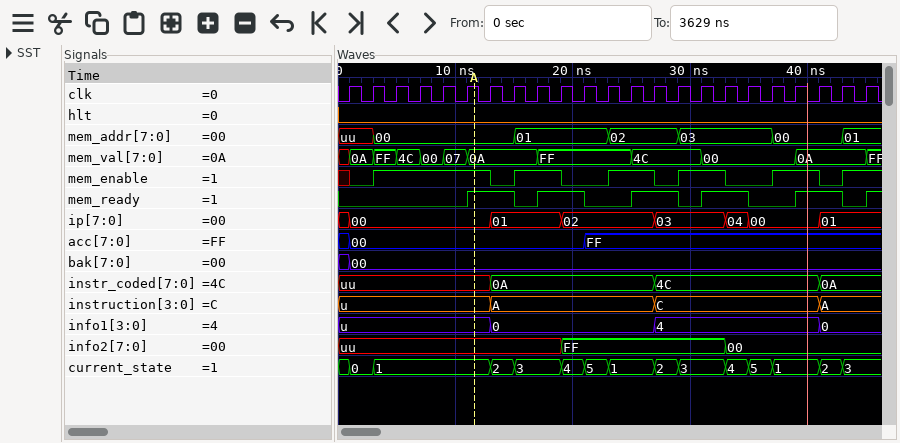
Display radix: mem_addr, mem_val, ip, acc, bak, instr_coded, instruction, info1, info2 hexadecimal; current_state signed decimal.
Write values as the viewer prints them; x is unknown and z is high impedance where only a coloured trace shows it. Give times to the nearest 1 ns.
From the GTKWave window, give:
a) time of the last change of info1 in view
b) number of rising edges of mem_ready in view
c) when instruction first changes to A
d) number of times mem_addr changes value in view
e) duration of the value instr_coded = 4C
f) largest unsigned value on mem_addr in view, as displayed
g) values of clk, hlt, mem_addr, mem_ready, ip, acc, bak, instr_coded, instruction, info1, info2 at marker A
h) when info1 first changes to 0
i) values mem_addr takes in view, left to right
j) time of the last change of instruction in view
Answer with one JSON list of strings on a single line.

["41 ns", "6", "13 ns", "6", "14 ns", "03", "clk=1, hlt=0, mem_addr=00, mem_ready=1, ip=00, acc=00, bak=00, instr_coded=uu, instruction=u, info1=u, info2=uu", "13 ns", "uu, 00, 01, 02, 03, 00, 01", "41 ns"]
